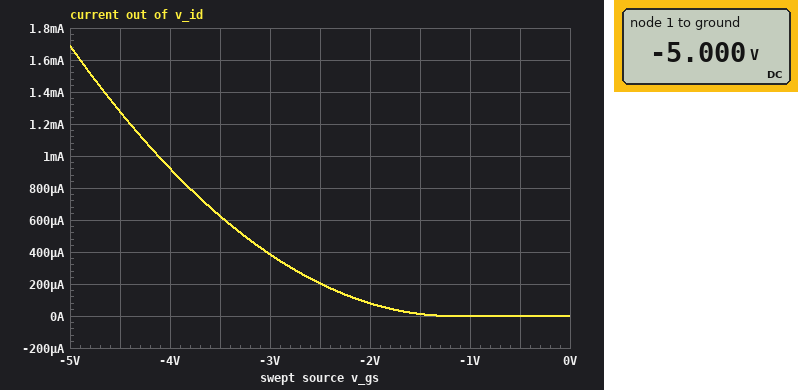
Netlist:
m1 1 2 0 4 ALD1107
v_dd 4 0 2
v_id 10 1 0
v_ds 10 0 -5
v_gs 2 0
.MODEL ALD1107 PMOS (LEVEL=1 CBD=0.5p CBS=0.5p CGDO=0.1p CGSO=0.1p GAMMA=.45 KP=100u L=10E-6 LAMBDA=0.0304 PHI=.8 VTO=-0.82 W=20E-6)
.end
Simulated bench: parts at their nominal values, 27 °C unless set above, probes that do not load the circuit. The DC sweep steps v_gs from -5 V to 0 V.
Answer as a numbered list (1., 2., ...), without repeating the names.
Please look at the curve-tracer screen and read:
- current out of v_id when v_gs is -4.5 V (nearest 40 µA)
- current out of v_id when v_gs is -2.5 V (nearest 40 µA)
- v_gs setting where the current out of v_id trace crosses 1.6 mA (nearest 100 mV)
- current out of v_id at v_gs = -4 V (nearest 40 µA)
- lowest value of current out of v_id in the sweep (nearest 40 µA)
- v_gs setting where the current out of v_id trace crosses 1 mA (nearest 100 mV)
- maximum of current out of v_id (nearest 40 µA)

1. 1.28 mA
2. 200 µA
3. -4.9 V
4. 920 µA
5. 0 A
6. -4.1 V
7. 1.68 mA
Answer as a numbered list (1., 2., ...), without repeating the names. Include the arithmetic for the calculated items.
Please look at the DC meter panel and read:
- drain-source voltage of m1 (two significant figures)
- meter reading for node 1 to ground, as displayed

1. -5 V = -5.0 V
2. -5.000 V
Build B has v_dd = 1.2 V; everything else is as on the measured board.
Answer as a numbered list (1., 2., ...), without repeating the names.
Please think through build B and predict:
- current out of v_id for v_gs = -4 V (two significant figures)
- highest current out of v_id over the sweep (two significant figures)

1. 1.0 mA
2. 1.8 mA
